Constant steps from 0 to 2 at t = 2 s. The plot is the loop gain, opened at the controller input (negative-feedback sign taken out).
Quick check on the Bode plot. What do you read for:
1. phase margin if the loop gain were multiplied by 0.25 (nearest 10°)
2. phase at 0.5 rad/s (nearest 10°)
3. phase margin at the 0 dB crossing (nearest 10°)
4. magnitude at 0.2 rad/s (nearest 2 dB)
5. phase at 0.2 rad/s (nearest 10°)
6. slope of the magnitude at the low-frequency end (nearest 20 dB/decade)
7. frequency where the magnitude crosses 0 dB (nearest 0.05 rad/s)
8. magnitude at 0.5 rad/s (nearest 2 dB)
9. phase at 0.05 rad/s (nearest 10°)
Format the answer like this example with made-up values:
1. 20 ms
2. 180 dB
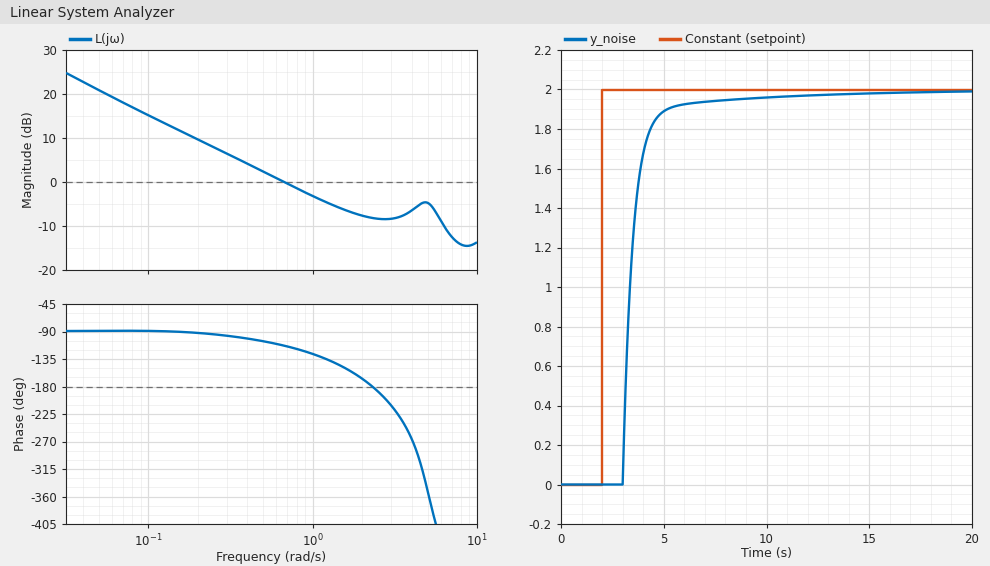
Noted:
1. 90°
2. -110°
3. 70°
4. 10 dB
5. -90°
6. -20 dB/decade
7. 0.65 rad/s
8. 2 dB
9. -90°
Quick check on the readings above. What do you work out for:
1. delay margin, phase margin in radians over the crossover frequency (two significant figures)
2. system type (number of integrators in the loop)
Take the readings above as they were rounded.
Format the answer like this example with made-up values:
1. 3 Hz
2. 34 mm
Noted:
1. 1.9 s
2. 1
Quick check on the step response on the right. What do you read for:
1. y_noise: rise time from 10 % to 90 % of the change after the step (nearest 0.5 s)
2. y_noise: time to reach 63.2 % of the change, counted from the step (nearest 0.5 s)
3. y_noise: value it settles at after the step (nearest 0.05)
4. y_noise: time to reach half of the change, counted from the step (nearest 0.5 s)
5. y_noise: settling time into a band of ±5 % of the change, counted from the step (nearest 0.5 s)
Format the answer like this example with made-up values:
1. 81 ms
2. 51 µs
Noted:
1. 1.5 s
2. 1.5 s
3. 2.00
4. 1.5 s
5. 3.0 s
